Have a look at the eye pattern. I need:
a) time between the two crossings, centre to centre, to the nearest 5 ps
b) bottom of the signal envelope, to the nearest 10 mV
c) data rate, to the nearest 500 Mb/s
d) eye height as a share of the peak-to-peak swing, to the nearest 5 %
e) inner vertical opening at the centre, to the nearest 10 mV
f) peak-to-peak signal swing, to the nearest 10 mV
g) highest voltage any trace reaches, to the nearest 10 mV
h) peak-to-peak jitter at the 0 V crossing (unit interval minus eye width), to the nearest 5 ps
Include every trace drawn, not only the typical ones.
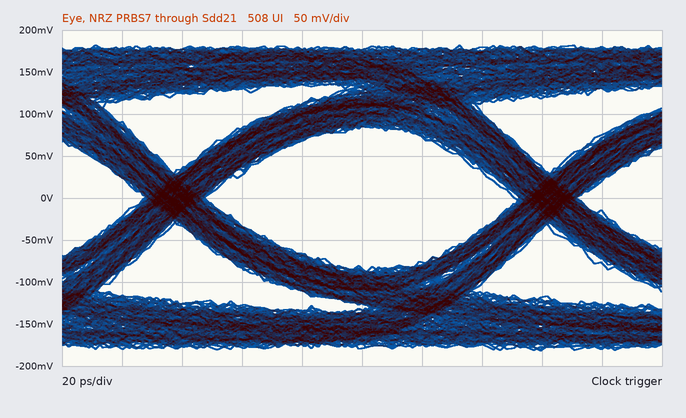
125 ps
-180 mV
8.0 Gb/s
45 %
170 mV
360 mV
180 mV
20 ps
